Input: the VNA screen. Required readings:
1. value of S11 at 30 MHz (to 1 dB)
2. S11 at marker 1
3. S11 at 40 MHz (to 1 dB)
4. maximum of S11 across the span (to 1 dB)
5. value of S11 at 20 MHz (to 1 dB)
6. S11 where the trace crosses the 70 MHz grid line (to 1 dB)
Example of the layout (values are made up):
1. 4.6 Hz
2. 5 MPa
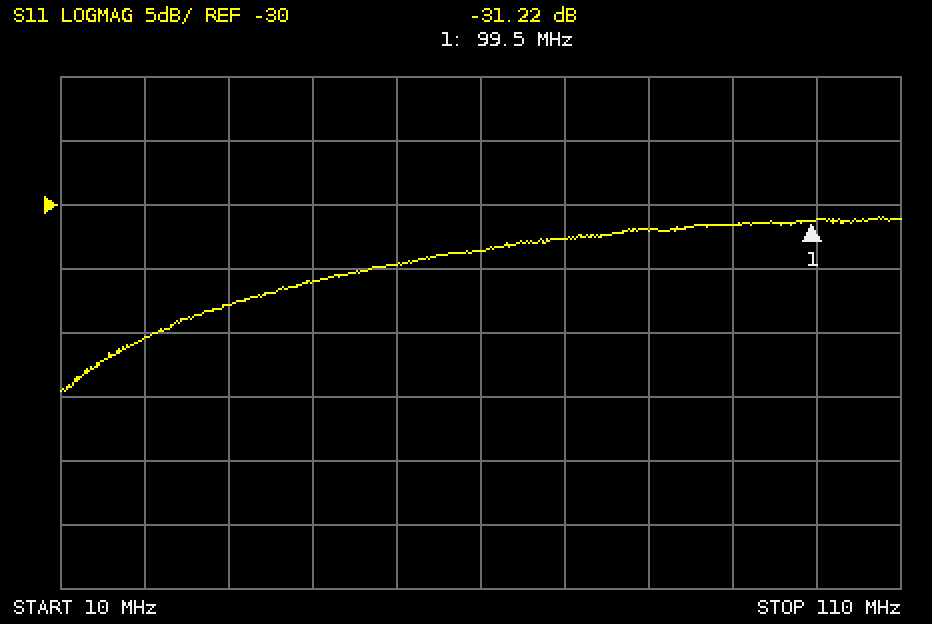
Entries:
1. -38 dB
2. -31.22 dB
3. -36 dB
4. -31 dB
5. -40 dB
6. -33 dB
